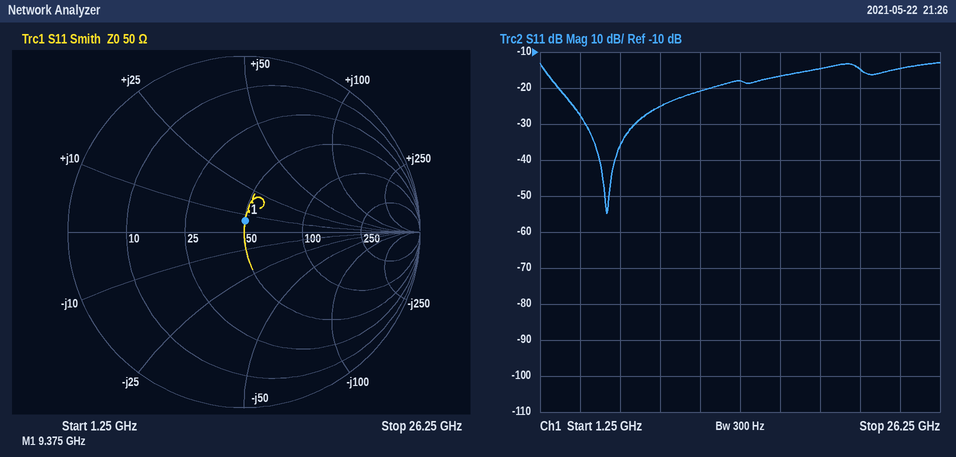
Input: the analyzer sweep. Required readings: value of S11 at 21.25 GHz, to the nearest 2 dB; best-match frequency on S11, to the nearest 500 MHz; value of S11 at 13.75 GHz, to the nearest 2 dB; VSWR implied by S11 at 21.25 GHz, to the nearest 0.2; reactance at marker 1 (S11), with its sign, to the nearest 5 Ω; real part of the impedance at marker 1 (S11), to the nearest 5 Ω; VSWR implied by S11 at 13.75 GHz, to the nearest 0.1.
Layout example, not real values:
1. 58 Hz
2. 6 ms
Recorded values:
1. -14 dB
2. 5.5 GHz
3. -18 dB
4. 1.4
5. +5 Ω
6. 50 Ω
7. 1.3
